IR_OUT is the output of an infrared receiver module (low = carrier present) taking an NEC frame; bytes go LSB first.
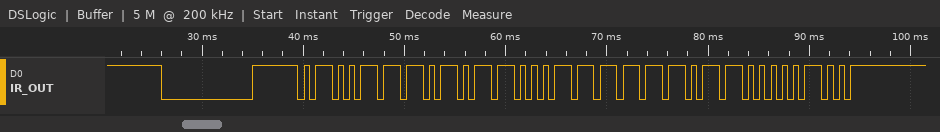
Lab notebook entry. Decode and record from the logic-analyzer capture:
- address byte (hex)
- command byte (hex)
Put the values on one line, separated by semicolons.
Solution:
0x72; 0xDF
